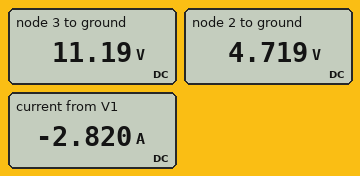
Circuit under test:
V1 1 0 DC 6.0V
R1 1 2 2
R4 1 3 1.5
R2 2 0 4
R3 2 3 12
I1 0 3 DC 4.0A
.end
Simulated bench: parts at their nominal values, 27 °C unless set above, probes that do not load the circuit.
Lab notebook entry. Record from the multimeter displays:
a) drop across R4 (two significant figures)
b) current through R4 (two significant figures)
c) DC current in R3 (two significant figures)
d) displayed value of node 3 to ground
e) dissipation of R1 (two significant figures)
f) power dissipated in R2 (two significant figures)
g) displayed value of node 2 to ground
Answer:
5.2 V
3.5 A
540 mA
11.19 V
820 mW
5.6 W
4.719 V
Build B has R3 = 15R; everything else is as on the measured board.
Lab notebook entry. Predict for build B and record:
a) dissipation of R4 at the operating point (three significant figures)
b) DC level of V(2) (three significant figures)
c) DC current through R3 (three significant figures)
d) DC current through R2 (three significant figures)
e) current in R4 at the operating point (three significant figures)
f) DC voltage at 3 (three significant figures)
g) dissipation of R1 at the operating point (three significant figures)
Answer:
18.9 W
4.60 V
449 mA
1.15 A
3.55 A
11.3 V
983 mW
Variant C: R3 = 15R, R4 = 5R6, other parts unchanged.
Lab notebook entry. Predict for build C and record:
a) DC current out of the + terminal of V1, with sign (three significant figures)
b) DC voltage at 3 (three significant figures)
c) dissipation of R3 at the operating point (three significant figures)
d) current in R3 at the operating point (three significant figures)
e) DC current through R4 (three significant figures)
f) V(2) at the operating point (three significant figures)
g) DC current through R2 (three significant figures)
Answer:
-2.63 A
22.2 V
18.6 W
1.11 A
2.89 A
5.48 V
1.37 A
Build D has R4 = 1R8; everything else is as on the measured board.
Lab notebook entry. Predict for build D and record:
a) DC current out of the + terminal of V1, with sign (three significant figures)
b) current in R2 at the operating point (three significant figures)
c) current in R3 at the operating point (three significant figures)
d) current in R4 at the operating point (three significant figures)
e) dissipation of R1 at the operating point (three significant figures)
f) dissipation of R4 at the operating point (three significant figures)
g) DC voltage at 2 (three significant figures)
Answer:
-2.80 A
1.20 A
608 mA
3.39 A
707 mW
20.7 W
4.81 V
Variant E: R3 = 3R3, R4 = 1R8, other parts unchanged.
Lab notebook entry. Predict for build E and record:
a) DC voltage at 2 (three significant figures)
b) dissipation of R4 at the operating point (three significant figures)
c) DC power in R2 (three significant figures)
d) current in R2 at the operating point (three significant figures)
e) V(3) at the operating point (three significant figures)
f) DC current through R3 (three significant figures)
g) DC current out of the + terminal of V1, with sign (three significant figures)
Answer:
5.91 V
11.9 W
8.72 W
1.48 A
10.6 V
1.43 A
-2.52 A
